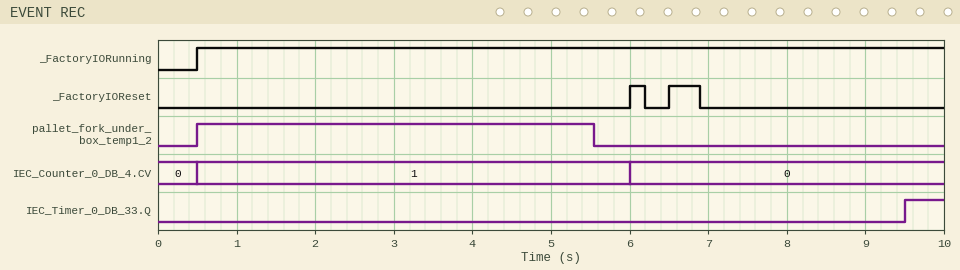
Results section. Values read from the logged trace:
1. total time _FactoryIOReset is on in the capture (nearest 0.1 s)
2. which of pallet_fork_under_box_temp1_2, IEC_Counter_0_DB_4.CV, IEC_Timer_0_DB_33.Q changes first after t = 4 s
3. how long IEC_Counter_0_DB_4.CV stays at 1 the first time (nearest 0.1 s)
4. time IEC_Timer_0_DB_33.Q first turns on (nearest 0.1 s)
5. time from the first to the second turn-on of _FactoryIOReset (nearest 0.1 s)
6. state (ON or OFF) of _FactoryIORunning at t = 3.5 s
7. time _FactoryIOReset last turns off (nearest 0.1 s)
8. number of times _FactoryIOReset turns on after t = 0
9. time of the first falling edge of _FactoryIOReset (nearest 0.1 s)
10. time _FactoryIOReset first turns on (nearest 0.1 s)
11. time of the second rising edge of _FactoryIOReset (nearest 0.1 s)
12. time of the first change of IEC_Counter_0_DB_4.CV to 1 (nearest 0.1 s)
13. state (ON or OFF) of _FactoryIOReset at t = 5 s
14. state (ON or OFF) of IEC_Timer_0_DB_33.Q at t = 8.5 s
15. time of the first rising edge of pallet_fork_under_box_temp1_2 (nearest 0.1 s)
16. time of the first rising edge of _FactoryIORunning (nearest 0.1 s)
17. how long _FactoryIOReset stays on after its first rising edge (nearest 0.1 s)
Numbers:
0.6 s
pallet_fork_under_box_temp1_2
5.5 s
9.5 s
0.5 s
ON
6.9 s
2
6.2 s
6.0 s
6.5 s
0.5 s
OFF
OFF
0.5 s
0.5 s
0.2 s
